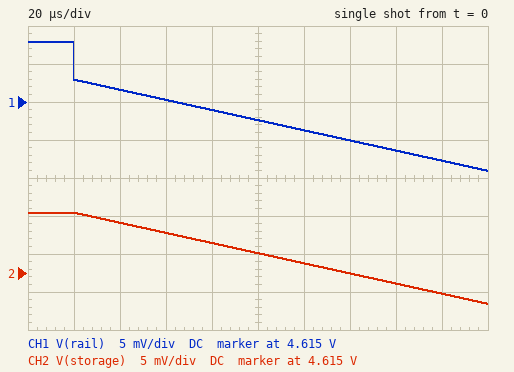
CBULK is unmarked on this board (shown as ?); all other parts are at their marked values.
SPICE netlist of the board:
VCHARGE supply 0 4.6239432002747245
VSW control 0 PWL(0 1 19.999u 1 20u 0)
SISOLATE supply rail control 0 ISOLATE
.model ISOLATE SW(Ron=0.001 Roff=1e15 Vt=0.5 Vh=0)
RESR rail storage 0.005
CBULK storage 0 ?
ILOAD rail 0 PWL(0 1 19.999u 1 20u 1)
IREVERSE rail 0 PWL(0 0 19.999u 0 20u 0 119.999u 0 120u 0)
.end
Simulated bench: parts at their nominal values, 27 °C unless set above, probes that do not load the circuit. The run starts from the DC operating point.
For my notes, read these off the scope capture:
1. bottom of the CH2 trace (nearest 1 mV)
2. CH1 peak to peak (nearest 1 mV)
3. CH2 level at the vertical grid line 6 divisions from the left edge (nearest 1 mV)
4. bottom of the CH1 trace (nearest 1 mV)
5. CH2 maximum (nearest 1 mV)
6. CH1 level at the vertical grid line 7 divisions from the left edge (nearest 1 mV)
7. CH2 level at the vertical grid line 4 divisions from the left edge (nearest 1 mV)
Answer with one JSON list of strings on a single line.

["4.611 V", "17 mV", "4.616 V", "4.606 V", "4.623 V", "4.610 V", "4.619 V"]
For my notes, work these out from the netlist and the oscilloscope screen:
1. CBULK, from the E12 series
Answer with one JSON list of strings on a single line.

["15 mF"]
